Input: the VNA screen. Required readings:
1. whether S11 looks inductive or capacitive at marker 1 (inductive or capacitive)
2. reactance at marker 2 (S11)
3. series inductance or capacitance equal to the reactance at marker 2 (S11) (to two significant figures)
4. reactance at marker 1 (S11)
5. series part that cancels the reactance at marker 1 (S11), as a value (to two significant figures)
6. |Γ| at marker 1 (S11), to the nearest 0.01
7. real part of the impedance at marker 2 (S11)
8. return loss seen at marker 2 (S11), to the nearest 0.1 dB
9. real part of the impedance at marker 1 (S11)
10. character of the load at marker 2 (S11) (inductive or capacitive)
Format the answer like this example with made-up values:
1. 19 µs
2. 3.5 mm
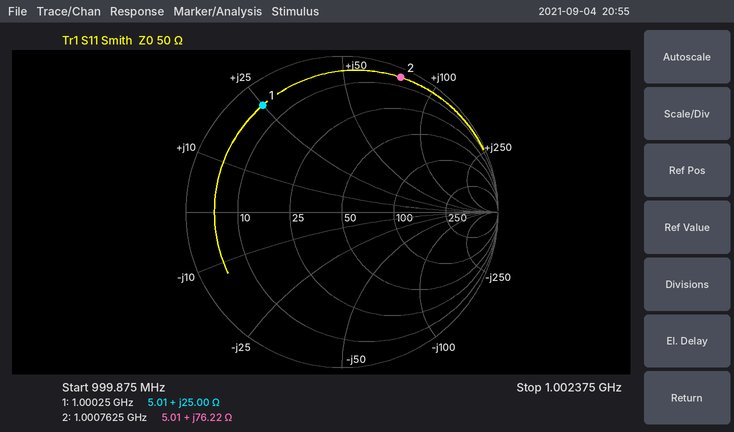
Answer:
1. inductive
2. +76.22 Ω
3. 12 nH
4. +25.00 Ω
5. 6.4 pF
6. 0.85
7. 5.01 Ω
8. 0.5 dB
9. 5.01 Ω
10. inductive
